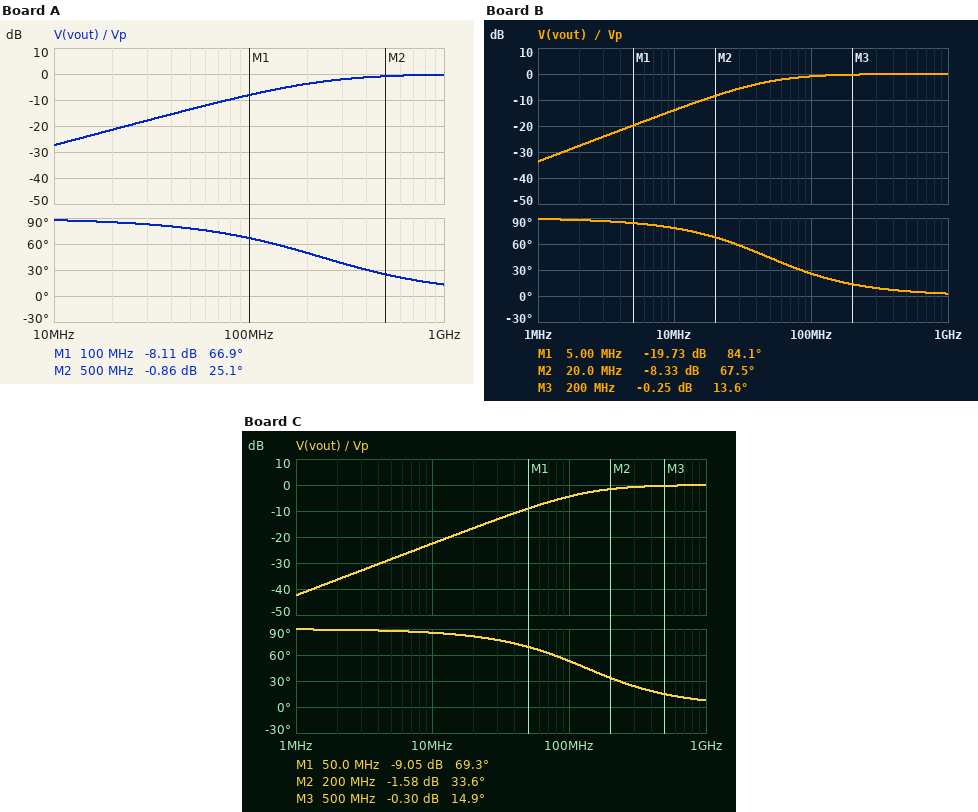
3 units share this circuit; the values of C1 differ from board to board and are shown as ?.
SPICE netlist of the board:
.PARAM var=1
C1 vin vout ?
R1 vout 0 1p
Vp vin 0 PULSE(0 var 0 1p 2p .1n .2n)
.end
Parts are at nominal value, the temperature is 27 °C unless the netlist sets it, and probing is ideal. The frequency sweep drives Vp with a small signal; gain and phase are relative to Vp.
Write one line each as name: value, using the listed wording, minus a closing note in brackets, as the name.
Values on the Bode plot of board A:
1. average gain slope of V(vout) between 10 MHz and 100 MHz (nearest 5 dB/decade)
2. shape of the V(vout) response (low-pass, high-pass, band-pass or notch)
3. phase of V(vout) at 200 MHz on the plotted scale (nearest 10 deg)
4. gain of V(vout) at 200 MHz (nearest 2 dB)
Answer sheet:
average gain slope of V(vout) between 10 MHz and 100 MHz: 20 dB/decade
shape of the V(vout) response: high-pass
phase of V(vout) at 200 MHz on the plotted scale: 50 deg
gain of V(vout) at 200 MHz: -4 dB
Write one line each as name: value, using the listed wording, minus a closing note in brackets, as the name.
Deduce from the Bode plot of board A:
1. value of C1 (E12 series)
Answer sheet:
value of C1: 680 F
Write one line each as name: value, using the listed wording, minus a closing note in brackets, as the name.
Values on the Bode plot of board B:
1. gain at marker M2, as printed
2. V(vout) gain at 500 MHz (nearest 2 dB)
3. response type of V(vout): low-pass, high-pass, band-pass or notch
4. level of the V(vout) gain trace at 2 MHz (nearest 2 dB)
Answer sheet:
gain at marker M2, as printed: -8.33 dB
V(vout) gain at 500 MHz: 0 dB
response type of V(vout): low-pass, high-pass, band-pass or notch: high-pass
level of the V(vout) gain trace at 2 MHz: -28 dB
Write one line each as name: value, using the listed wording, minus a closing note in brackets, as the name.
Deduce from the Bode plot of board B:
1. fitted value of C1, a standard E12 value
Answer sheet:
fitted value of C1, a standard E12 value: 3.3 kF
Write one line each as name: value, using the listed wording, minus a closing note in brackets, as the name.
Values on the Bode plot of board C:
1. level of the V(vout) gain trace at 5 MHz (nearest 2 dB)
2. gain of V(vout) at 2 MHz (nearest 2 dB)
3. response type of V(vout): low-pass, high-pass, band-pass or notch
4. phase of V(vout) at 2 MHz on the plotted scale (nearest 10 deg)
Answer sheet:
level of the V(vout) gain trace at 5 MHz: -28 dB
gain of V(vout) at 2 MHz: -36 dB
response type of V(vout): low-pass, high-pass, band-pass or notch: high-pass
phase of V(vout) at 2 MHz on the plotted scale: 90 deg
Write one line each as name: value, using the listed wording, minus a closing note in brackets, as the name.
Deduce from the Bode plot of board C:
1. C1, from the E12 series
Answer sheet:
C1, from the E12 series: 1.2 kF
